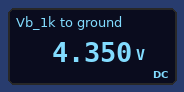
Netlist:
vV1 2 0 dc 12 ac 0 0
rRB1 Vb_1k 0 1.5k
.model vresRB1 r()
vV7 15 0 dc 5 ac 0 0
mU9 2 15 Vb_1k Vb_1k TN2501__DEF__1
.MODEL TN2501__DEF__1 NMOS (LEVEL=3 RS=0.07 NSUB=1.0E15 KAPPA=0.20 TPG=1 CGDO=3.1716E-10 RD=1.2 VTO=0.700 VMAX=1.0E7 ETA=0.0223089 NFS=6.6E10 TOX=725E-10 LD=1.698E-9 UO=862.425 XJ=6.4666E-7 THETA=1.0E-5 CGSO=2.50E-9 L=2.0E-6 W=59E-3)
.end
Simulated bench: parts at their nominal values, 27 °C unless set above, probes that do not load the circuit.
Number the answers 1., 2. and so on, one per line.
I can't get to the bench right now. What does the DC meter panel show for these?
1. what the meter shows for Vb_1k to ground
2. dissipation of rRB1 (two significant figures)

1. 4.350 V
2. 13 mW
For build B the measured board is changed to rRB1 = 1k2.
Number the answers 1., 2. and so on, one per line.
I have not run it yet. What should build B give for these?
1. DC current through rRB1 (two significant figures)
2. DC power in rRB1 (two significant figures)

1. 3.6 mA
2. 16 mW
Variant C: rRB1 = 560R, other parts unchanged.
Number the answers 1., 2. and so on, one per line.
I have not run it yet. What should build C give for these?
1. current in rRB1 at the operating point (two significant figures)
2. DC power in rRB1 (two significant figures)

1. 7.7 mA
2. 33 mW
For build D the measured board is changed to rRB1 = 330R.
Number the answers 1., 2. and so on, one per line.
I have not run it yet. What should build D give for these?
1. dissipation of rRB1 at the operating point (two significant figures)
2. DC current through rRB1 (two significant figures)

1. 55 mW
2. 13 mA
